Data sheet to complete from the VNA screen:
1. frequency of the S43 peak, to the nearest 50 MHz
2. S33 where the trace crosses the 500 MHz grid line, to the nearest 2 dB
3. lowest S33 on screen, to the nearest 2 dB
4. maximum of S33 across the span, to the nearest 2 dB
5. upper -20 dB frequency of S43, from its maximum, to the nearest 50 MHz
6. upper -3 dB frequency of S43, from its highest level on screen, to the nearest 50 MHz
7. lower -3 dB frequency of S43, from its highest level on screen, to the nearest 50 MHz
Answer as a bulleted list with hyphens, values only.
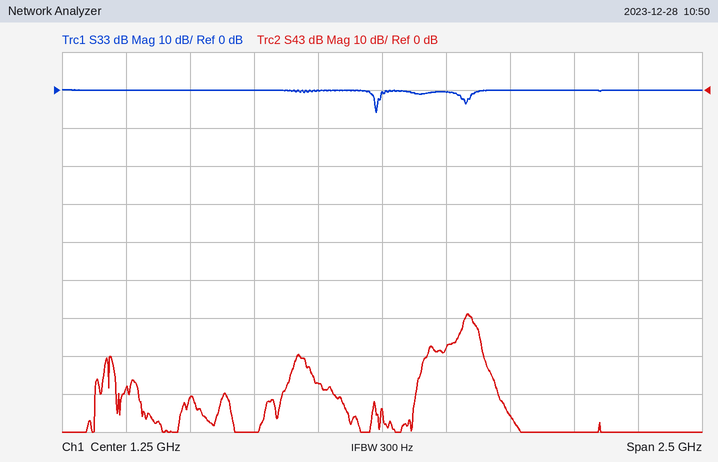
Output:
- 1.60 GHz
- 0 dB
- -6 dB
- 0 dB
- 1.70 GHz
- 1.60 GHz
- 1.55 GHz
